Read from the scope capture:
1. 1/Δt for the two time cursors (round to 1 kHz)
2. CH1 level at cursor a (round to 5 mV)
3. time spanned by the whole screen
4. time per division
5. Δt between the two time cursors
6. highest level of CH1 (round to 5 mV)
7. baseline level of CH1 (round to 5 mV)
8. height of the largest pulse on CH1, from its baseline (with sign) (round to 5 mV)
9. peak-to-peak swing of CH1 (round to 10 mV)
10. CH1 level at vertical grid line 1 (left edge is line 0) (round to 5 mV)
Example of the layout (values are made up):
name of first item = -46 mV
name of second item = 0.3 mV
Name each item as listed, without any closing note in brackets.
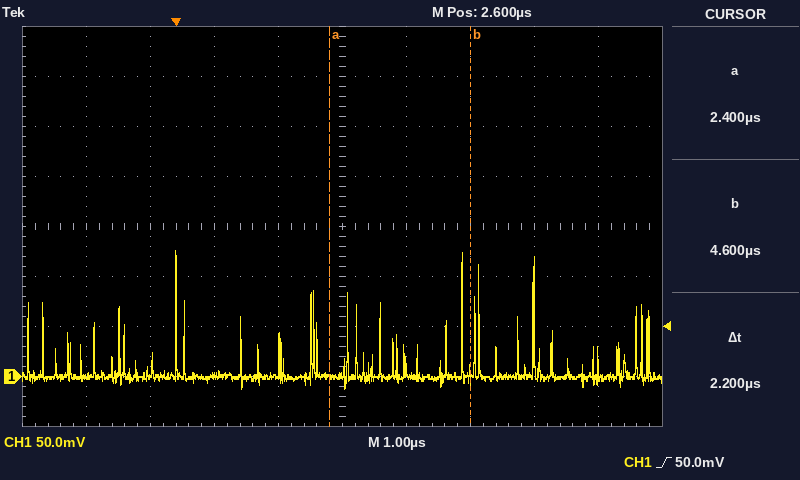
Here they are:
1/Δt for the two time cursors = 455 kHz
CH1 level at cursor a = 0 mV
time spanned by the whole screen = 10 µs
time per division = 1 µs
Δt between the two time cursors = 2.2 µs
highest level of CH1 = 125 mV
baseline level of CH1 = 0 mV
height of the largest pulse on CH1, from its baseline (with sign) = +125 mV
peak-to-peak swing of CH1 = 140 mV
CH1 level at vertical grid line 1 (left edge is line 0) = 0 mV
